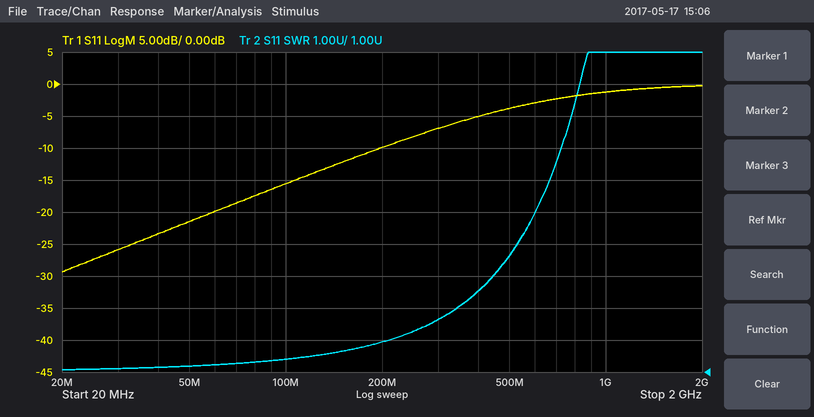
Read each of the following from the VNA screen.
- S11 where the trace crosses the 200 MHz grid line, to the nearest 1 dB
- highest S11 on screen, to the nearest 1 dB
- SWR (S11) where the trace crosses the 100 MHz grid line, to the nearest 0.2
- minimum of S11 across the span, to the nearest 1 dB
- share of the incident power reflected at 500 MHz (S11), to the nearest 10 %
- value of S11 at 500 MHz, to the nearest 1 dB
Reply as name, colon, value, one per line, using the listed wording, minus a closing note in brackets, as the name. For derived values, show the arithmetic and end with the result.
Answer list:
S11 where the trace crosses the 200 MHz grid line, to the nearest 1 dB: -10 dB
highest S11 on screen, to the nearest 1 dB: 0 dB
SWR (S11) where the trace crosses the 100 MHz grid line, to the nearest 0.2: 1.4
minimum of S11 across the span, to the nearest 1 dB: -29 dB
share of the incident power reflected at 500 MHz (S11), to the nearest 10 %: 10^(-4/10) ≈ 40 %
value of S11 at 500 MHz, to the nearest 1 dB: -4 dB
